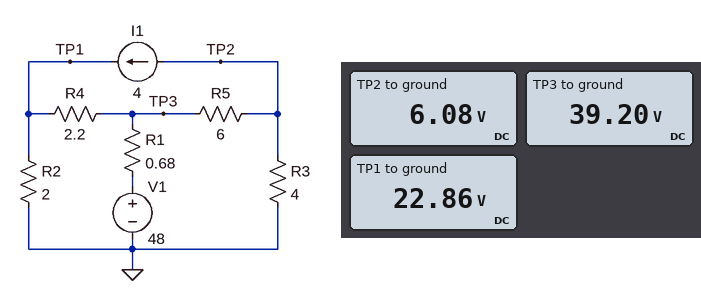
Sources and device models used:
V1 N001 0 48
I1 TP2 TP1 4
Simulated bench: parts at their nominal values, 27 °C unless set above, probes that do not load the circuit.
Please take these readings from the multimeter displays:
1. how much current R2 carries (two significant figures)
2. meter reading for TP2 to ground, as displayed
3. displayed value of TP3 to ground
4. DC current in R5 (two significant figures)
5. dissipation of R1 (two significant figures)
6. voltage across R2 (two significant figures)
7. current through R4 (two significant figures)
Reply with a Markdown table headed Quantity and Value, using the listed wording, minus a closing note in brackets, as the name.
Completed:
| Quantity | Value |
|---|---|
| how much current R2 carries | 11 A |
| meter reading for TP2 to ground, as displayed | 6.08 V |
| displayed value of TP3 to ground | 39.20 V |
| DC current in R5 | 5.5 A |
| dissipation of R1 | 110 W |
| voltage across R2 | 23 V |
| current through R4 | 7.4 A |
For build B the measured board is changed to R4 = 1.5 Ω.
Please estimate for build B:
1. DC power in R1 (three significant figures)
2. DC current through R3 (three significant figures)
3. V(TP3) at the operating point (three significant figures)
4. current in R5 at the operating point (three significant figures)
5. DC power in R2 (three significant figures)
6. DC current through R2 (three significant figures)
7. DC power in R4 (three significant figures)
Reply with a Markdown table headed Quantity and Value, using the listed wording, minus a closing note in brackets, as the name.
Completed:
| Quantity | Value |
|---|---|
| DC power in R1 | 136 W |
| DC current through R3 | 1.44 A |
| V(TP3) at the operating point | 38.4 V |
| current in R5 at the operating point | 5.44 A |
| DC power in R2 | 322 W |
| DC current through R2 | 12.7 A |
| DC power in R4 | 113 W |
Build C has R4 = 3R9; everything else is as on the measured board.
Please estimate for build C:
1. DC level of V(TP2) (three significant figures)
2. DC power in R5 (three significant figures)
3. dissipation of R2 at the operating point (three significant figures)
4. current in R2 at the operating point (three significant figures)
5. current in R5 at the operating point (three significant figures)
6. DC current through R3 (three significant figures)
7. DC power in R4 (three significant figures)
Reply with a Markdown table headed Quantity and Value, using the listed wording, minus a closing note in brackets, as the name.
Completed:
| Quantity | Value |
|---|---|
| DC level of V(TP2) | 6.57 V |
| DC power in R5 | 191 W |
| dissipation of R2 at the operating point | 180 W |
| current in R2 at the operating point | 9.50 A |
| current in R5 at the operating point | 5.64 A |
| DC current through R3 | 1.64 A |
| DC power in R4 | 118 W |
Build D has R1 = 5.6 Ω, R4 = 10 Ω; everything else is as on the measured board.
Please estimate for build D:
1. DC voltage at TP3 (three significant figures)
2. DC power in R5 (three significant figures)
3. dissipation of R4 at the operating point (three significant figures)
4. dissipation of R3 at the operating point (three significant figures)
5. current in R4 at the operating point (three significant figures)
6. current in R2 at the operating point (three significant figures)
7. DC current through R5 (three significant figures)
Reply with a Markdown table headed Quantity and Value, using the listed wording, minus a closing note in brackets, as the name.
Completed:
| Quantity | Value |
|---|---|
| DC voltage at TP3 | 21.1 V |
| DC power in R5 | 82.6 W |
| dissipation of R4 at the operating point | 11.9 W |
| dissipation of R3 at the operating point | 335 mW |
| current in R4 at the operating point | 1.09 A |
| current in R2 at the operating point | 5.09 A |
| DC current through R5 | 3.71 A |
